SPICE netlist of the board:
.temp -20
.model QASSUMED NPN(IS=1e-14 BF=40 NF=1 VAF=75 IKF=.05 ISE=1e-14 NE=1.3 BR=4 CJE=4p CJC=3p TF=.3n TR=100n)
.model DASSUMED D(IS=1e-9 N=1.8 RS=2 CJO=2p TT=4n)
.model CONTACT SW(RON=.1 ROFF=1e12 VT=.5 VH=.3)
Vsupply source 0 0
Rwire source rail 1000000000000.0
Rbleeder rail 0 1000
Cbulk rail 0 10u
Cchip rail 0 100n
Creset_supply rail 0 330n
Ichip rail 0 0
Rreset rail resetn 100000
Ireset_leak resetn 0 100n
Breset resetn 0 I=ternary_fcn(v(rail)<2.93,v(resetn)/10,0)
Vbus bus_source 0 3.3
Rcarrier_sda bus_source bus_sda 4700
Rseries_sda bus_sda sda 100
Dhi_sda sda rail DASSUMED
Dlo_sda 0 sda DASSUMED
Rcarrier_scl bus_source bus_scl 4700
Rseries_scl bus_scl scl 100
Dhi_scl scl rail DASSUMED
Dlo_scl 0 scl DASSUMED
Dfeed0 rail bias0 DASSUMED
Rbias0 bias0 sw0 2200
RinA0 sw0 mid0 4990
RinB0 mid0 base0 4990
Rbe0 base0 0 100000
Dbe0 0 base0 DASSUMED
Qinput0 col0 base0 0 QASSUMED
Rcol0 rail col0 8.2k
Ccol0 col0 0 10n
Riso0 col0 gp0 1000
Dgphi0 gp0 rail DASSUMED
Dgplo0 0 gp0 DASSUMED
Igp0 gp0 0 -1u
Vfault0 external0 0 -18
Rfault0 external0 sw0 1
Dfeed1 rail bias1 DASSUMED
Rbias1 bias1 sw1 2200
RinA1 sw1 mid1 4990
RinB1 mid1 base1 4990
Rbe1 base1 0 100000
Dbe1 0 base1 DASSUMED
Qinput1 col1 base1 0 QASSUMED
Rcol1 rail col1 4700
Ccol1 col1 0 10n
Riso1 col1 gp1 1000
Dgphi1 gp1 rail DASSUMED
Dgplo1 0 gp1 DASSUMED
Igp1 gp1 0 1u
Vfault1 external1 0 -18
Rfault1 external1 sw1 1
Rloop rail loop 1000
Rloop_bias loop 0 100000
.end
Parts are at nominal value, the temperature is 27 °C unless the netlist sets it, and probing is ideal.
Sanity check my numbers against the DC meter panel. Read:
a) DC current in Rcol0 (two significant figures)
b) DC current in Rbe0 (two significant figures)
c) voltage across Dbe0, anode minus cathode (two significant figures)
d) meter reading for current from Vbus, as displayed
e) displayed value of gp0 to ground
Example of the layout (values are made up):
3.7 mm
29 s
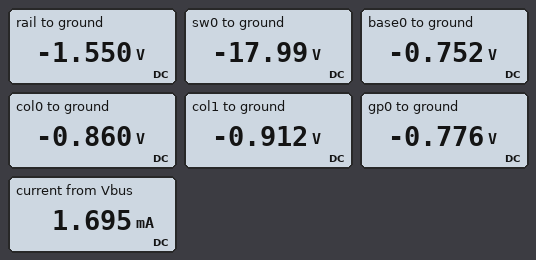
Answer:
84 µA
7.5 µA
750 mV
1.695 mA
-0.776 V
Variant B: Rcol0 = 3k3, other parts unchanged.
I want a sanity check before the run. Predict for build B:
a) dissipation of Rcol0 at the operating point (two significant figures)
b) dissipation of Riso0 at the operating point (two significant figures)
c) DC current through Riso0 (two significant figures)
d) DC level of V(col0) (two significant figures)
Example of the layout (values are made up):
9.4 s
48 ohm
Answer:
110 µW
32 µW
180 µA
-960 mV
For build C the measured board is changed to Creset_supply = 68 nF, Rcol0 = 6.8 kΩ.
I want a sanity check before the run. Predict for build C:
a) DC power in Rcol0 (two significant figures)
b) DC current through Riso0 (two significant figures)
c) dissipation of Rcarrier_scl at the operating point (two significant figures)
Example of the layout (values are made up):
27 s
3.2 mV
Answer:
67 µW
99 µA
3.4 mW
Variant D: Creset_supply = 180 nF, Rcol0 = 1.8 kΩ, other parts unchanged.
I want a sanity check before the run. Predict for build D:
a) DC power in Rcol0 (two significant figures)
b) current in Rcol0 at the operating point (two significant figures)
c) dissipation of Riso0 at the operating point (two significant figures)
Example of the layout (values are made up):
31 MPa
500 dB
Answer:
140 µW
280 µA
76 µW
